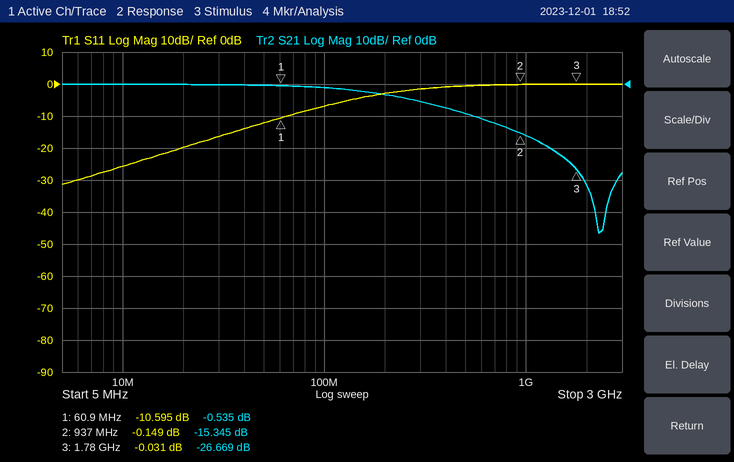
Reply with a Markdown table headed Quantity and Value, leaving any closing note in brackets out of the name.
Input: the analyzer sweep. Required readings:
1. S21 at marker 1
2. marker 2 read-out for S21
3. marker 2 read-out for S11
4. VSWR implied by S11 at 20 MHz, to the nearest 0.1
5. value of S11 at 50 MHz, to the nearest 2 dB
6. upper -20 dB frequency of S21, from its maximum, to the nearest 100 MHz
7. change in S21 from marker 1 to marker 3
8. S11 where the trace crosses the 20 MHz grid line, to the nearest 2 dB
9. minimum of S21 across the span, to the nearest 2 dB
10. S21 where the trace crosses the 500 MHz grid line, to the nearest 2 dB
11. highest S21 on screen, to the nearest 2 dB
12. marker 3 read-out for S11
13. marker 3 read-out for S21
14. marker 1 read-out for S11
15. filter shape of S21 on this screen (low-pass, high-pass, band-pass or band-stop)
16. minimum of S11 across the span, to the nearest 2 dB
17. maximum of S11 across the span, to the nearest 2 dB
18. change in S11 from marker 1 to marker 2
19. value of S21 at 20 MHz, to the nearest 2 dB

| Quantity | Value |
|---|---|
| S21 at marker 1 | -0.535 dB |
| marker 2 read-out for S21 | -15.345 dB |
| marker 2 read-out for S11 | -0.149 dB |
| VSWR implied by S11 at 20 MHz, to the nearest 0.1 | 1.2 |
| value of S11 at 50 MHz, to the nearest 2 dB | -12 dB |
| upper -20 dB frequency of S21, from its maximum, to the nearest 100 MHz | 1.3 GHz |
| change in S21 from marker 1 to marker 3 | -26.134 dB |
| S11 where the trace crosses the 20 MHz grid line, to the nearest 2 dB | -20 dB |
| minimum of S21 across the span, to the nearest 2 dB | -46 dB |
| S21 where the trace crosses the 500 MHz grid line, to the nearest 2 dB | -10 dB |
| highest S21 on screen, to the nearest 2 dB | 0 dB |
| marker 3 read-out for S11 | -0.031 dB |
| marker 3 read-out for S21 | -26.669 dB |
| marker 1 read-out for S11 | -10.595 dB |
| filter shape of S21 on this screen | low-pass |
| minimum of S11 across the span, to the nearest 2 dB | -32 dB |
| maximum of S11 across the span, to the nearest 2 dB | 0 dB |
| change in S11 from marker 1 to marker 2 | 10.446 dB |
| value of S21 at 20 MHz, to the nearest 2 dB | 0 dB |
